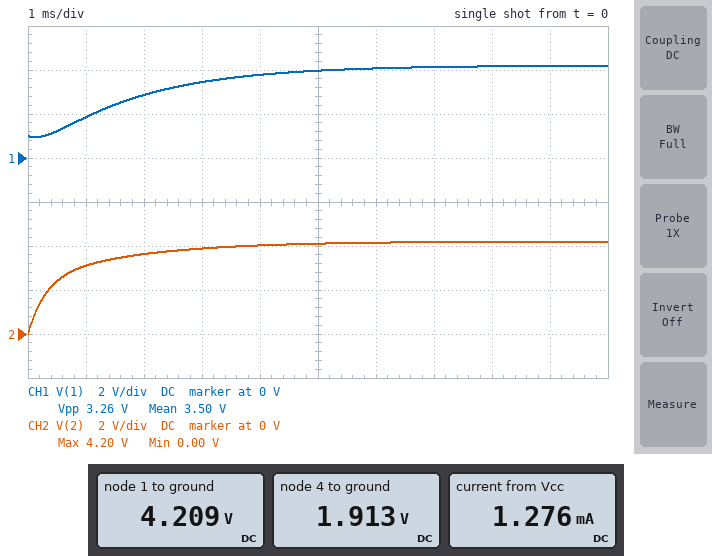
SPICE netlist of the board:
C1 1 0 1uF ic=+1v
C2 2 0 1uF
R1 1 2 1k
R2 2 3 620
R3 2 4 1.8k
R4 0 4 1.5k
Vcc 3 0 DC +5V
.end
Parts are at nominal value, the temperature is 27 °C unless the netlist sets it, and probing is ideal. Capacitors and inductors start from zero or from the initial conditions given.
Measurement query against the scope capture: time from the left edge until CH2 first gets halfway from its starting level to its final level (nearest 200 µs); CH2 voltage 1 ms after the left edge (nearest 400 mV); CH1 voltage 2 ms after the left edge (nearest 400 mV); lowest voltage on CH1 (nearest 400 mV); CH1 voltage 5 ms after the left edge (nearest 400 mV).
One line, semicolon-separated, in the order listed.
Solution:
400 µs; 3.2 V; 2.8 V; 800 mV; 4.0 V
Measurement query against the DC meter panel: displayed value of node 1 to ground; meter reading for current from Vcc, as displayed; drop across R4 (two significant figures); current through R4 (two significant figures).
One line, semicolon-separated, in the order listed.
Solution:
4.209 V; 1.276 mA; 1.9 V; 1.3 mA
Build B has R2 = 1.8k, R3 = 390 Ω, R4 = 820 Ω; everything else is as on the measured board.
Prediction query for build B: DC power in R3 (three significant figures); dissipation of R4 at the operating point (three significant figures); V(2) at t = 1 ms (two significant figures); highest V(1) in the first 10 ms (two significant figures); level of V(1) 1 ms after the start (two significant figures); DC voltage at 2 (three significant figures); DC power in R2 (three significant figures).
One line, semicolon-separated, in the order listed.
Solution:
1.08 mW; 2.26 mW; 1.4 V; 2.0 V; 1.0 V; 2.01 V; 4.97 mW
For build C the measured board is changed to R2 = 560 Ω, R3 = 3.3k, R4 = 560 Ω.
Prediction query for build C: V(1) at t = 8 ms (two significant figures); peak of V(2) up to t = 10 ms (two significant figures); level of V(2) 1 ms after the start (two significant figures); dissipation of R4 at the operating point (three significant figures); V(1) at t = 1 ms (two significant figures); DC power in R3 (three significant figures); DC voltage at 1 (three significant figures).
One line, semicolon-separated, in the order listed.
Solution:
4.3 V; 4.4 V; 3.3 V; 717 µW; 2.0 V; 4.22 mW; 4.37 V
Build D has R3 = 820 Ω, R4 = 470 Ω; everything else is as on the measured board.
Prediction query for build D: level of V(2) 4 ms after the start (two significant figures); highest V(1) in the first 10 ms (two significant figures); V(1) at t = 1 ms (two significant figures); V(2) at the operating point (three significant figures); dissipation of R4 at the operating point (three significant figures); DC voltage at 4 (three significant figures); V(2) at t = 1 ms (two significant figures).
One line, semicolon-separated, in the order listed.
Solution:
3.3 V; 3.4 V; 1.7 V; 3.38 V; 3.22 mW; 1.23 V; 2.7 V
